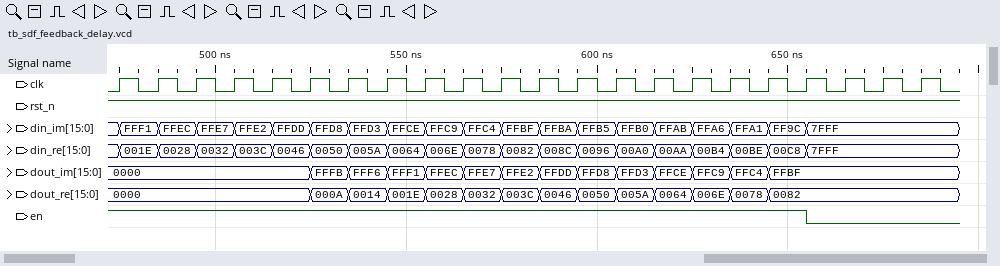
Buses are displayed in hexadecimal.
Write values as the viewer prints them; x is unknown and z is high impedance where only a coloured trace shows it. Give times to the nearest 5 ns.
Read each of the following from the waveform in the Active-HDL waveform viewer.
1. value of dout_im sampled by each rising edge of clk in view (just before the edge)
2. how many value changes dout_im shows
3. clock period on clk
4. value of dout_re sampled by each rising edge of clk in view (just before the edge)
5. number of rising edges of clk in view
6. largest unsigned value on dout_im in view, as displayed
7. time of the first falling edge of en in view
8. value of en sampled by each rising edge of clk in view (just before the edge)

0000, 0000, 0000, 0000, 0000, 0000, FFFB, FFF6, FFF1, FFEC, FFE7, FFE2, FFDD, FFD8, FFD3, FFCE, FFC9, FFC4, FFBF, FFBF, FFBF, FFBF
13
10 ns
0000, 0000, 0000, 0000, 0000, 0000, 000A, 0014, 001E, 0028, 0032, 003C, 0046, 0050, 005A, 0064, 006E, 0078, 0082, 0082, 0082, 0082
22
FFFB
655 ns
1 1 1 1 1 1 1 1 1 1 1 1 1 1 1 1 1 1 1 0 0 0
